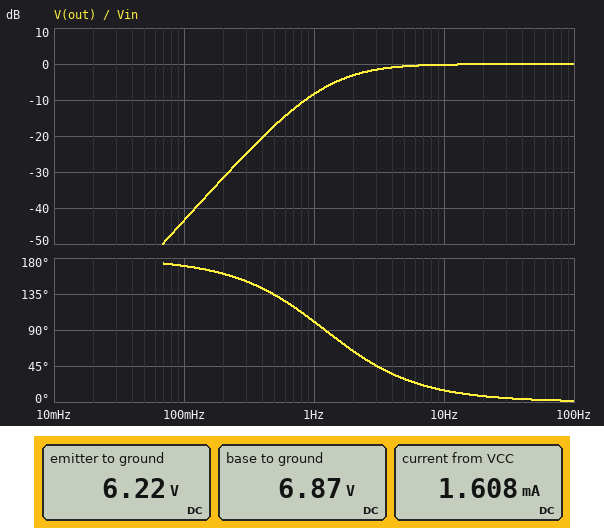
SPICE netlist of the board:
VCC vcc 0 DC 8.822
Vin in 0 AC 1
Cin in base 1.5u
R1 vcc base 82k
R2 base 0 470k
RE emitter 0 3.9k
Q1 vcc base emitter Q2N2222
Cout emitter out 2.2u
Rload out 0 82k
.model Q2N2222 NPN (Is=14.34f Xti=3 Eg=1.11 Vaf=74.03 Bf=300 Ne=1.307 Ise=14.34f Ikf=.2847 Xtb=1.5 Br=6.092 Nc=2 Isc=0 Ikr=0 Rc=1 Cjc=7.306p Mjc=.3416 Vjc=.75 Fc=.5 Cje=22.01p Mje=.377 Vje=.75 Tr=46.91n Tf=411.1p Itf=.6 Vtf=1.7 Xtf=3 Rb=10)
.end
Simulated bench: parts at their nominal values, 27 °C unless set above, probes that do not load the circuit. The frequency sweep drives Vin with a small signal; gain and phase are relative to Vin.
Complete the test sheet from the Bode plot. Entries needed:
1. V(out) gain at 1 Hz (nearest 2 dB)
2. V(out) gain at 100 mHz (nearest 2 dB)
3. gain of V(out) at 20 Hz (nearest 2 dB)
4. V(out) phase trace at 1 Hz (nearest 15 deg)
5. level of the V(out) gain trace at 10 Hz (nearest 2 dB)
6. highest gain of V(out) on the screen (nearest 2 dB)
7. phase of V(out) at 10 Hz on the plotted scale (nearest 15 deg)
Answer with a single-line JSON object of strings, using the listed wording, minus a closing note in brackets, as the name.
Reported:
{"V(out) gain at 1 Hz": "-8 dB", "V(out) gain at 100 mHz": "-44 dB", "gain of V(out) at 20 Hz": "0 dB", "V(out) phase trace at 1 Hz": "105 deg", "level of the V(out) gain trace at 10 Hz": "0 dB", "highest gain of V(out) on the screen": "0 dB", "phase of V(out) at 10 Hz on the plotted scale": "15 deg"}
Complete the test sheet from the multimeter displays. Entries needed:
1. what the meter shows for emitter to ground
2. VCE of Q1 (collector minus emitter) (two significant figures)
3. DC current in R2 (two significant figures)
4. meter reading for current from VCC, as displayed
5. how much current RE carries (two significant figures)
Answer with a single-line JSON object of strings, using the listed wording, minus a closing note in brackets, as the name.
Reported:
{"what the meter shows for emitter to ground": "6.22 V", "VCE of Q1 (collector minus emitter)": "2.6 V", "DC current in R2": "15 µA", "meter reading for current from VCC, as displayed": "1.608 mA", "how much current RE carries": "1.6 mA"}
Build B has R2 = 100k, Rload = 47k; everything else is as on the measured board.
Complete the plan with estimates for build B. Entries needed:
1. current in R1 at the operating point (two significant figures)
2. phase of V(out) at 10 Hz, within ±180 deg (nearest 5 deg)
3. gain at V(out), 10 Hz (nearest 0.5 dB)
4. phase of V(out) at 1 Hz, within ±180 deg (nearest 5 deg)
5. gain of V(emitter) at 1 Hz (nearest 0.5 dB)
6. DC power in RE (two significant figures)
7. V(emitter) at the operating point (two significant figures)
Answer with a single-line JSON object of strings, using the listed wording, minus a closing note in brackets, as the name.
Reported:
{"current in R1 at the operating point": "52 µA", "phase of V(out) at 10 Hz, within ±180 deg": "25 deg", "gain at V(out), 10 Hz": "-0.5 dB", "phase of V(out) at 1 Hz, within ±180 deg": "125 deg", "gain of V(emitter) at 1 Hz": "-8.5 dB", "DC power in RE": "4.0 mW", "V(emitter) at the operating point": "3.9 V"}
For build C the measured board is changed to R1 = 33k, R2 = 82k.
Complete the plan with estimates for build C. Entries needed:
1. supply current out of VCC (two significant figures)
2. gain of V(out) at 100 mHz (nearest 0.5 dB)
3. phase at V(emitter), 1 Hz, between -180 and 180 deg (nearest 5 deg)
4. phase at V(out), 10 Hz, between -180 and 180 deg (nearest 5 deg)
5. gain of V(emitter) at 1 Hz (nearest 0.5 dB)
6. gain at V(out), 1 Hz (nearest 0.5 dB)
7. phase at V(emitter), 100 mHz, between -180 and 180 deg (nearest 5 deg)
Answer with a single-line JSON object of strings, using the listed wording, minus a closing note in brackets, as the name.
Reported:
{"supply current out of VCC": "1.5 mA", "gain of V(out) at 100 mHz": "-52.5 dB", "phase at V(emitter), 1 Hz, between -180 and 180 deg": "80 deg", "phase at V(out), 10 Hz, between -180 and 180 deg": "30 deg", "gain of V(emitter) at 1 Hz": "-13.5 dB", "gain at V(out), 1 Hz": "-16.0 dB", "phase at V(emitter), 100 mHz, between -180 and 180 deg": "90 deg"}
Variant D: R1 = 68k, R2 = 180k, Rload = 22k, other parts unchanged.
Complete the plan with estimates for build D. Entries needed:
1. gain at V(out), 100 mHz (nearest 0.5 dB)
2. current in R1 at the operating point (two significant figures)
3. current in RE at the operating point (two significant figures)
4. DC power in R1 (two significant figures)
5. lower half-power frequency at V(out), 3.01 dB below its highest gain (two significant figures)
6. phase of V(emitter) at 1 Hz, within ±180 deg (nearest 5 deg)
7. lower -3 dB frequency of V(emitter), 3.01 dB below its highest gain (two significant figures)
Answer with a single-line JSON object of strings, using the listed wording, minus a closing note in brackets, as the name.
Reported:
{"gain at V(out), 100 mHz": "-57.5 dB", "current in R1 at the operating point": "41 µA", "current in RE at the operating point": "1.4 mA", "DC power in R1": "120 µW", "lower half-power frequency at V(out), 3.01 dB below its highest gain": "4.4 Hz", "phase of V(emitter) at 1 Hz, within ±180 deg": "65 deg", "lower -3 dB frequency of V(emitter), 3.01 dB below its highest gain": "2.3 Hz"}
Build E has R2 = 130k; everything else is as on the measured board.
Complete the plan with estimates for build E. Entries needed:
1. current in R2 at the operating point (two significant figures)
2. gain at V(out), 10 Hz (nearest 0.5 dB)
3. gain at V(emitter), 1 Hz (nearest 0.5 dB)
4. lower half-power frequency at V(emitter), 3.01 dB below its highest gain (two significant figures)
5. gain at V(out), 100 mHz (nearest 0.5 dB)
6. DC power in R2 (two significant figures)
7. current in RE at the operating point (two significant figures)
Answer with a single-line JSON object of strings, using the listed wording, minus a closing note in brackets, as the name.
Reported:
{"current in R2 at the operating point": "39 µA", "gain at V(out), 10 Hz": "-0.5 dB", "gain at V(emitter), 1 Hz": "-8.0 dB", "lower half-power frequency at V(emitter), 3.01 dB below its highest gain": "2.3 Hz", "gain at V(out), 100 mHz": "-46.0 dB", "DC power in R2": "200 µW", "current in RE at the operating point": "1.1 mA"}
